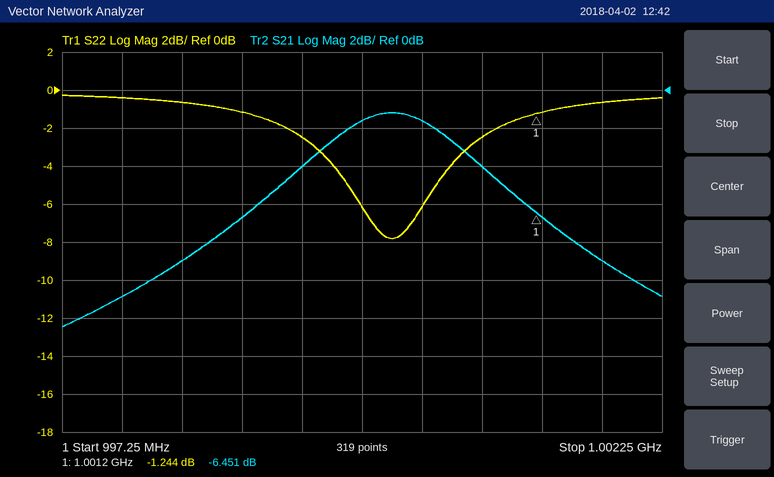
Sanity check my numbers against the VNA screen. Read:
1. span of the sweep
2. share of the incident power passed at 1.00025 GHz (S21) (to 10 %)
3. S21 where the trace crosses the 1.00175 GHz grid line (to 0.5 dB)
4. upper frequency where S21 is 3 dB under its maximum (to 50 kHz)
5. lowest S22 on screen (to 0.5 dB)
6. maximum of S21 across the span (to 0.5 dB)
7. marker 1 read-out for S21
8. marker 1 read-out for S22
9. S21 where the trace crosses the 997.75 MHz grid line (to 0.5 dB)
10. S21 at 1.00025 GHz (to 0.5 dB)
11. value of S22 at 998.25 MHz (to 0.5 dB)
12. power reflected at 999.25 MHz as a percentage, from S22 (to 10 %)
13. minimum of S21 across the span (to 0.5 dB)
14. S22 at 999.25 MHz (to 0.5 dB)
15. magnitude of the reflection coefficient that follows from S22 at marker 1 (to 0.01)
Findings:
5 MHz
70 %
-9.0 dB
1.00080 GHz
-8.0 dB
-1.0 dB
-6.451 dB
-1.244 dB
-11.0 dB
-1.5 dB
-0.5 dB
60 %
-12.5 dB
-2.5 dB
0.87
